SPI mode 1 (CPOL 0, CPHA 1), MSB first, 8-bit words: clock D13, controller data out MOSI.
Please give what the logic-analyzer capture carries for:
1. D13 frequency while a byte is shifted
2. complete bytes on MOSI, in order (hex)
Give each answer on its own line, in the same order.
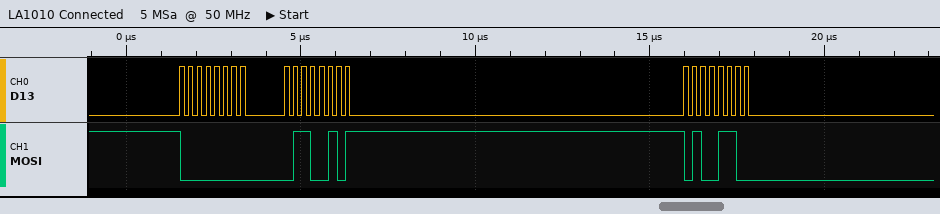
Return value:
4 MHz
00 65 4C
